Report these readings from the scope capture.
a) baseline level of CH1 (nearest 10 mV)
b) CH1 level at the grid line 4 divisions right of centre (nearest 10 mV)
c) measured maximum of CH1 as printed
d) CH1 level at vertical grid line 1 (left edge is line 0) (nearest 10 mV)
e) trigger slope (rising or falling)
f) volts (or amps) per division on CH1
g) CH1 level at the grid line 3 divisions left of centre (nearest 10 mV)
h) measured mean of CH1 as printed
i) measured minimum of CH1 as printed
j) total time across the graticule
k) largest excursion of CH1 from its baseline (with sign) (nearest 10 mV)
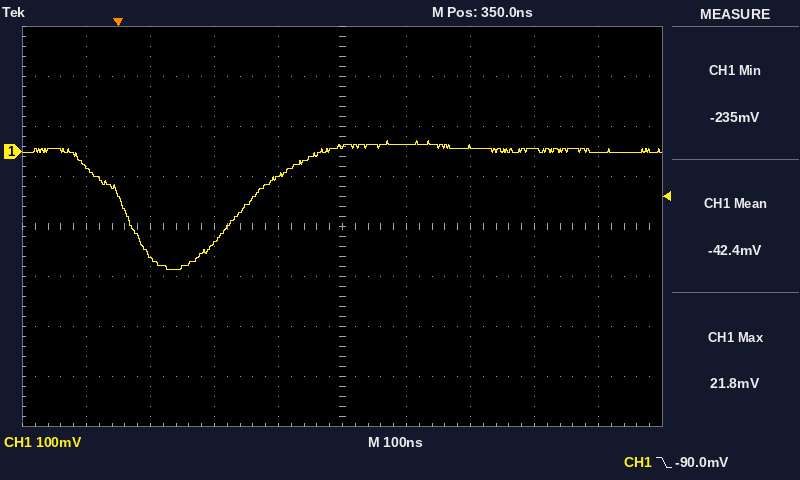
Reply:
0 mV
0 mV
21.8 mV
-30 mV
falling
100 mV
-210 mV
-42.4 mV
-235 mV
1 µs
-240 mV
